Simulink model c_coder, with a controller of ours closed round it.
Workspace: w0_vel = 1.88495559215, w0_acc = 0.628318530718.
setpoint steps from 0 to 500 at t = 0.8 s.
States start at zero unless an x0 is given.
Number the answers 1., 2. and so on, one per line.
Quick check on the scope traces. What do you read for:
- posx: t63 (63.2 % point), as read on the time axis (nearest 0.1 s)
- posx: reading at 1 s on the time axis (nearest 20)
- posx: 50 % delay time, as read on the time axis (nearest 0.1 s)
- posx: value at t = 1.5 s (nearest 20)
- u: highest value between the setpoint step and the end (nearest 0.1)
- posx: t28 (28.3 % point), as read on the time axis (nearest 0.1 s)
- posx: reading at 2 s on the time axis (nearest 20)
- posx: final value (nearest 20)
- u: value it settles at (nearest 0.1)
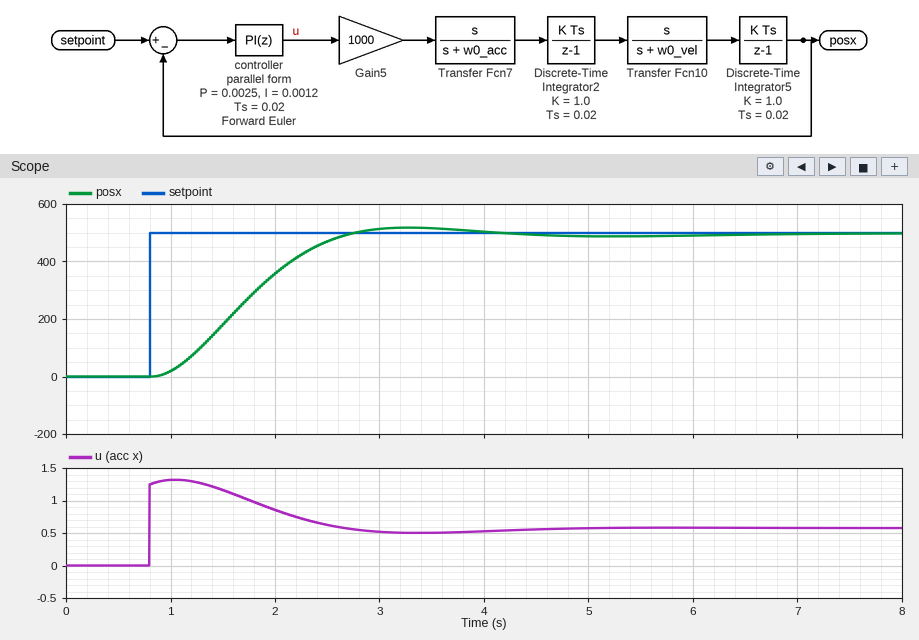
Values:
1. 1.9 s
2. 20
3. 1.7 s
4. 180
5. 1.3
6. 1.4 s
7. 360
8. 500
9. 0.6
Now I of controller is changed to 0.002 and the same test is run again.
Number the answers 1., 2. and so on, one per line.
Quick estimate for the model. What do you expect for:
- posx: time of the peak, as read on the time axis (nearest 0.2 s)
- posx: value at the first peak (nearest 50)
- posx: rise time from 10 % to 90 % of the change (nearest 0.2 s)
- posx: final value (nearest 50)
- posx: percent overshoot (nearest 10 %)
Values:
1. 3.2 s
2. 600
3. 1.0 s
4. 500
5. 20 %
